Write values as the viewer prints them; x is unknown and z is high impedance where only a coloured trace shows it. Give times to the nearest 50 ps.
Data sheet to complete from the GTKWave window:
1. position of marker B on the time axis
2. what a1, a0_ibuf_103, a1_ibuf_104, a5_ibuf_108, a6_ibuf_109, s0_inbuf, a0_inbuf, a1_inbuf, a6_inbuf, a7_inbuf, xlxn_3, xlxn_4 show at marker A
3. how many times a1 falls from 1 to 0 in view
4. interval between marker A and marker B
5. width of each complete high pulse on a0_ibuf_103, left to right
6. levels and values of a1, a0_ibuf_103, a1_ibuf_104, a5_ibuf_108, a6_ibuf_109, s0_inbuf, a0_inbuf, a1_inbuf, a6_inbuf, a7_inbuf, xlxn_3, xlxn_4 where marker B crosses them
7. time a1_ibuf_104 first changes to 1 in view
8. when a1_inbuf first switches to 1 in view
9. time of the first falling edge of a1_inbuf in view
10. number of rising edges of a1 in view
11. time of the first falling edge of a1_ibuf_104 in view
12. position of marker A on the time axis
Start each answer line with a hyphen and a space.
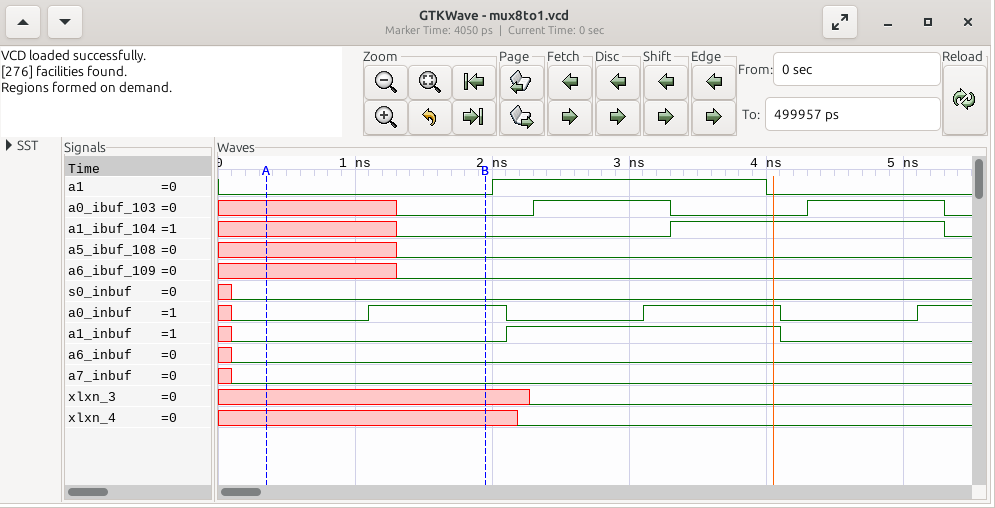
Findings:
- 1950 ps
- a1=0, a0_ibuf_103=x, a1_ibuf_104=x, a5_ibuf_108=x, a6_ibuf_109=x, s0_inbuf=0, a0_inbuf=0, a1_inbuf=0, a6_inbuf=0, a7_inbuf=0, xlxn_3=x, xlxn_4=x
- 1
- 1600 ps
- 1000 ps, 1000 ps
- a1=0, a0_ibuf_103=0, a1_ibuf_104=0, a5_ibuf_108=0, a6_ibuf_109=0, s0_inbuf=0, a0_inbuf=1, a1_inbuf=0, a6_inbuf=0, a7_inbuf=0, xlxn_3=x, xlxn_4=x
- 3300 ps
- 2100 ps
- 4100 ps
- 1
- 5300 ps
- 350 ps
